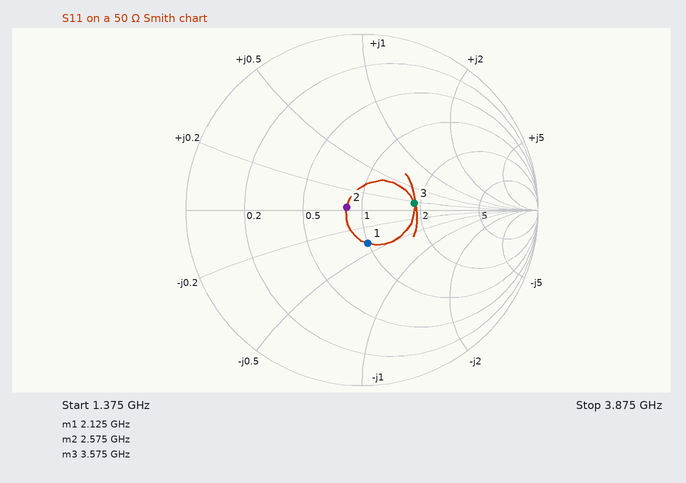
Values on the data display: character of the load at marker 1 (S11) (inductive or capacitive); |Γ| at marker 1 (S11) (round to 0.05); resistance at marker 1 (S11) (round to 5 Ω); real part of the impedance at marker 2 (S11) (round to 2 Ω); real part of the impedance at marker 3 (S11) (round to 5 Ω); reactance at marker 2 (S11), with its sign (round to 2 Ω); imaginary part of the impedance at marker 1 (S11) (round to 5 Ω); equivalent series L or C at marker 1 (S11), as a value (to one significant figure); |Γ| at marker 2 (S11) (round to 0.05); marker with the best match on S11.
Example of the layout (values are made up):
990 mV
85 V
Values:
capacitive
0.20
50 Ω
42 Ω
90 Ω
+2 Ω
-20 Ω
4 pF
0.10
marker 2
